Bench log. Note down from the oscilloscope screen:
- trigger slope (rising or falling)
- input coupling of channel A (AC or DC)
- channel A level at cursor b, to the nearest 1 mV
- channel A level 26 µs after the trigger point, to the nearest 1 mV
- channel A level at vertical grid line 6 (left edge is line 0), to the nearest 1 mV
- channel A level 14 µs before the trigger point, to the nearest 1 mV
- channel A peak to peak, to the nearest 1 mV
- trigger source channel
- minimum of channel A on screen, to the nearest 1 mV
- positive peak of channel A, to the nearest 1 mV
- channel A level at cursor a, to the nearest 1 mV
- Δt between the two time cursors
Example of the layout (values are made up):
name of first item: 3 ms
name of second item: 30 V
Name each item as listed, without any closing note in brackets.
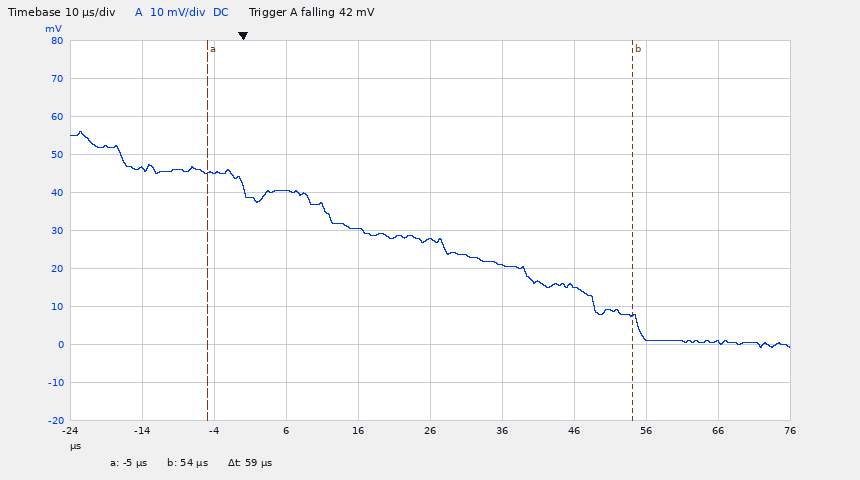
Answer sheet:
trigger slope: falling
input coupling of channel A: DC
channel A level at cursor b, to the nearest 1 mV: 7 mV
channel A level 26 µs after the trigger point, to the nearest 1 mV: 28 mV
channel A level at vertical grid line 6 (left edge is line 0), to the nearest 1 mV: 21 mV
channel A level 14 µs before the trigger point, to the nearest 1 mV: 46 mV
channel A peak to peak, to the nearest 1 mV: 57 mV
trigger source channel: channel A
minimum of channel A on screen, to the nearest 1 mV: -1 mV
positive peak of channel A, to the nearest 1 mV: 56 mV
channel A level at cursor a, to the nearest 1 mV: 45 mV
Δt between the two time cursors: 59 µs
